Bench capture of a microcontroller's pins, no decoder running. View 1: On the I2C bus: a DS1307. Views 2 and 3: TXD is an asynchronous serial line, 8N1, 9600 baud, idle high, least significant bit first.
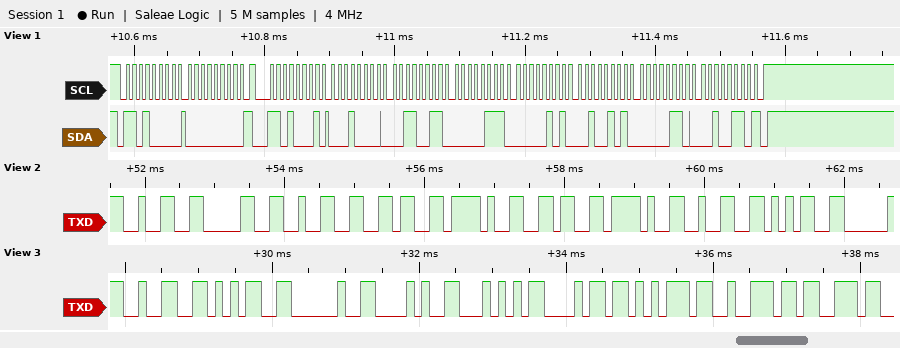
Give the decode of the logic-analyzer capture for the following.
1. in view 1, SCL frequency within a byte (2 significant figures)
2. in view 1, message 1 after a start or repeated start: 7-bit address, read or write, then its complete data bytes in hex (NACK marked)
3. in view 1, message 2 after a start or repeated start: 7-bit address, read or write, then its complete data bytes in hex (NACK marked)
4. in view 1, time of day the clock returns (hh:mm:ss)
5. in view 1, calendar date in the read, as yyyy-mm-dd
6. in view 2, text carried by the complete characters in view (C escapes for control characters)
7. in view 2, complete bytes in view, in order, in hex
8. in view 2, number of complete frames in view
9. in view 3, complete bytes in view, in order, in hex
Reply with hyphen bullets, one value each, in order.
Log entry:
- 100 kHz
- 0x68 write: 00
- 0x68 read: 10 33 07 05 25 06 26 NACK
- 07:33:10
- 2026-06-25
- "2026/6/25"
- 32 30 32 36 2F 36 2F 32 35
- 9
- 32 35 20 28 54 68 75 72 73
